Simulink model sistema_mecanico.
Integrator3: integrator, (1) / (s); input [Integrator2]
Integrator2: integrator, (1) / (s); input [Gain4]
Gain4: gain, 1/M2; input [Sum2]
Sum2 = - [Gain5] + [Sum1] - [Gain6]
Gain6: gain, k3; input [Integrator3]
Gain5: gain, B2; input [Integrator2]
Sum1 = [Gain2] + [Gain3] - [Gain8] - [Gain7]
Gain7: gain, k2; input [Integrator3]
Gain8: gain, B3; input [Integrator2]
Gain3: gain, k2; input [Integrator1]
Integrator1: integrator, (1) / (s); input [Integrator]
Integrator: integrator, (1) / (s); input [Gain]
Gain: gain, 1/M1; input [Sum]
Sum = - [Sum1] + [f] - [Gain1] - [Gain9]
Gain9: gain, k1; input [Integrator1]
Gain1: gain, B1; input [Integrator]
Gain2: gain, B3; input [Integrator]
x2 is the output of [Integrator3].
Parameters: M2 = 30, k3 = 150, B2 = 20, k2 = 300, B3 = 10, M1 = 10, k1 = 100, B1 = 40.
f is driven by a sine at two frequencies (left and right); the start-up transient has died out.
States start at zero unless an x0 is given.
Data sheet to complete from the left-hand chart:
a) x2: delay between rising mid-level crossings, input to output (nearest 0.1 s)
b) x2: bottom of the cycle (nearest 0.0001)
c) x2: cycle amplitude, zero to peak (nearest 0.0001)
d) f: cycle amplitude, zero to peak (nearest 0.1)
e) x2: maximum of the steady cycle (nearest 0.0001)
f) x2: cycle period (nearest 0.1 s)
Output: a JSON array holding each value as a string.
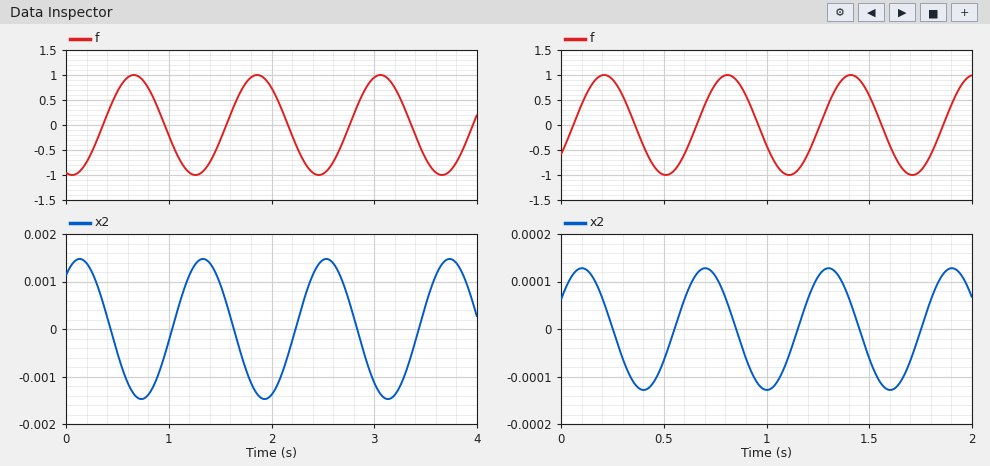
["0.7 s", "-0.0015", "0.0015", "1.0", "0.0015", "1.2 s"]
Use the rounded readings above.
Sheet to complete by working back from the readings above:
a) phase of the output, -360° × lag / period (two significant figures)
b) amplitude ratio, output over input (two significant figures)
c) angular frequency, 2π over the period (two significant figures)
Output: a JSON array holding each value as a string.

["-210°", "0.0015", "5.2 rad/s"]
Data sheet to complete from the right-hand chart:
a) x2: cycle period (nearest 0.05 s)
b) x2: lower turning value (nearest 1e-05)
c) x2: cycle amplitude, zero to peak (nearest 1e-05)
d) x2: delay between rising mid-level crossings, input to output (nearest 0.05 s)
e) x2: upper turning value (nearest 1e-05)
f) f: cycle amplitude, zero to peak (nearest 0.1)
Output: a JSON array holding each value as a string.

["0.60 s", "-0.00013", "0.00013", "0.50 s", "0.00013", "1.0"]
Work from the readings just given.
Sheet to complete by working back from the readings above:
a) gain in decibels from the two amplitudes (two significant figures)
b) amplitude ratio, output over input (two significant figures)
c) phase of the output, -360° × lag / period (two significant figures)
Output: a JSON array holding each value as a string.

["-78 dB", "0.00013", "-300°"]
